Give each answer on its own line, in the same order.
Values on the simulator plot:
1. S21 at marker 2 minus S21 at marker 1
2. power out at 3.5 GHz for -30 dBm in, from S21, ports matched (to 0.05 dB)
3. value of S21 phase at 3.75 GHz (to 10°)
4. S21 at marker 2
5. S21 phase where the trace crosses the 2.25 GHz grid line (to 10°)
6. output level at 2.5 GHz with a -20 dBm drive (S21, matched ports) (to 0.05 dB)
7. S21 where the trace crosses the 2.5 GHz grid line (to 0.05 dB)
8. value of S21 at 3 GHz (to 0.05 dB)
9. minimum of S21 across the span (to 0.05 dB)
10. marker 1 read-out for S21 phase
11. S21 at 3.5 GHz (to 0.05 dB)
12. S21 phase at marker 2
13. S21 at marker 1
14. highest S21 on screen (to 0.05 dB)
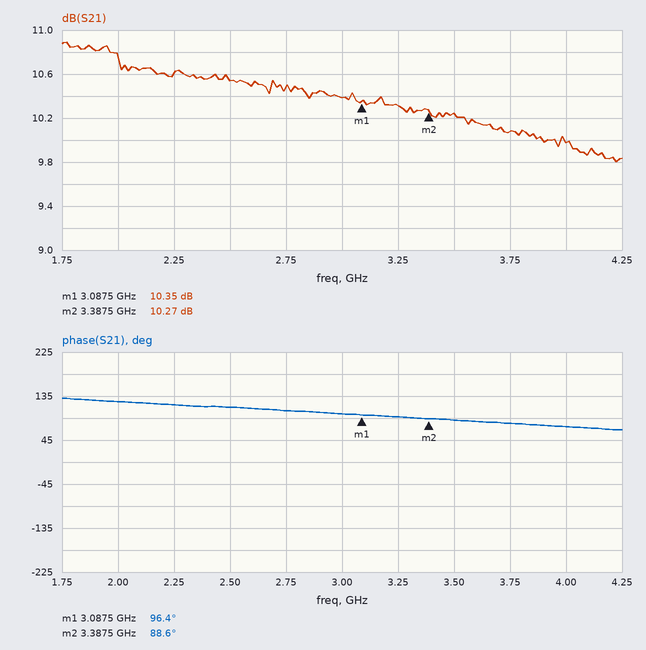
-0.08 dB
-19.75 dBm
80°
10.27 dB
120°
-9.45 dBm
10.55 dB
10.40 dB
9.80 dB
96.4°
10.25 dB
88.6°
10.35 dB
10.90 dB
